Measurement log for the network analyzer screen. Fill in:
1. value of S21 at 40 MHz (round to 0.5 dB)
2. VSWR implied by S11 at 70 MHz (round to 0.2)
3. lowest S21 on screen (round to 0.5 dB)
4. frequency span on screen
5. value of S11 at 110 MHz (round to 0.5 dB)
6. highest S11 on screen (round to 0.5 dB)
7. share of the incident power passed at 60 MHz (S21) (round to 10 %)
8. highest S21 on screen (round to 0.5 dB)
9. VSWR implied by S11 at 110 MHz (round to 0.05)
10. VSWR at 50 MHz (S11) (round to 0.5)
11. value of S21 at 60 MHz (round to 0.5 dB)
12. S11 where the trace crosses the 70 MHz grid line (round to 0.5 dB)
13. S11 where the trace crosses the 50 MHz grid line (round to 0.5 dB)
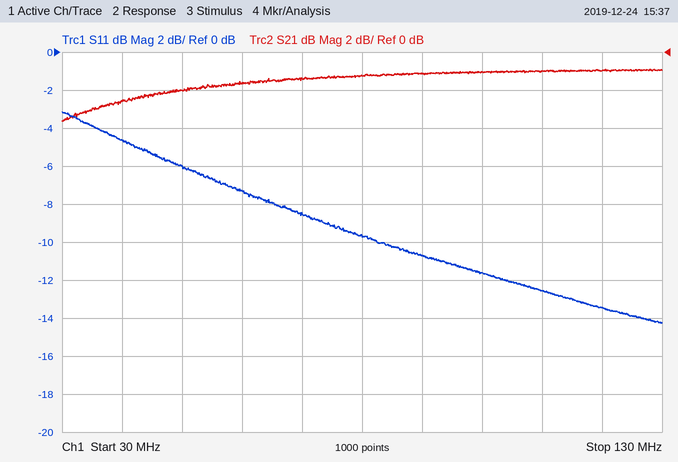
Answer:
-2.5 dB
2.2
-3.5 dB
100 MHz
-12.5 dB
-3.0 dB
70 %
-1.0 dB
1.60
3.0
-1.5 dB
-8.5 dB
-6.0 dB
